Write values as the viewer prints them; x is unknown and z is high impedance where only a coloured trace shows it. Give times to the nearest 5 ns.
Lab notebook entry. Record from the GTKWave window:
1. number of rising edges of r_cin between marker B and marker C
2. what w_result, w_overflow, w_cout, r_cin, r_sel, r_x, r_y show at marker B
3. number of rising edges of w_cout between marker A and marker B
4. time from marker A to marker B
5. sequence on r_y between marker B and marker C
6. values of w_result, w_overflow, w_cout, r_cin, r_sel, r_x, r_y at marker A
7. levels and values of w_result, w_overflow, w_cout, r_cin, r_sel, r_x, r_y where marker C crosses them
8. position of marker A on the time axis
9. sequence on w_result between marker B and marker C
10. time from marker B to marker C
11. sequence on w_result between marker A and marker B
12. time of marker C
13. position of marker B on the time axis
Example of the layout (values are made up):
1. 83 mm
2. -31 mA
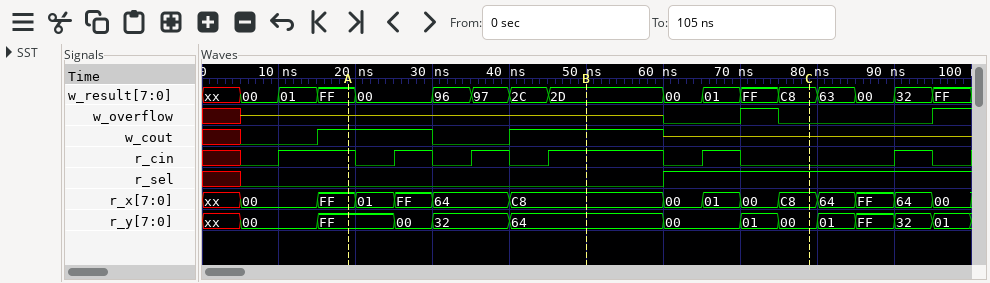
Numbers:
1. 1
2. w_result=2D, w_overflow=z, w_cout=1, r_cin=1, r_sel=0, r_x=C8, r_y=64
3. 1
4. 30 ns
5. 64, 00, 01, 00
6. w_result=FF, w_overflow=z, w_cout=1, r_cin=1, r_sel=0, r_x=FF, r_y=FF
7. w_result=C8, w_overflow=0, w_cout=z, r_cin=0, r_sel=1, r_x=C8, r_y=00
8. 20 ns
9. 2D, 00, 01, FF, C8
10. 30 ns
11. FF, 00, 96, 97, 2C, 2D
12. 80 ns
13. 50 ns
